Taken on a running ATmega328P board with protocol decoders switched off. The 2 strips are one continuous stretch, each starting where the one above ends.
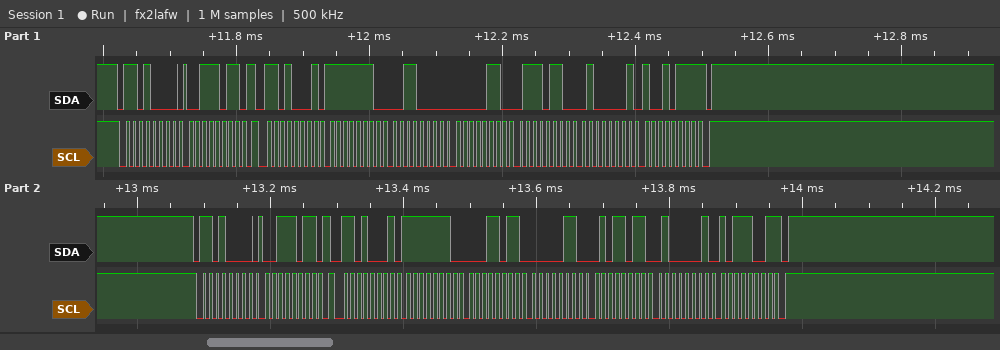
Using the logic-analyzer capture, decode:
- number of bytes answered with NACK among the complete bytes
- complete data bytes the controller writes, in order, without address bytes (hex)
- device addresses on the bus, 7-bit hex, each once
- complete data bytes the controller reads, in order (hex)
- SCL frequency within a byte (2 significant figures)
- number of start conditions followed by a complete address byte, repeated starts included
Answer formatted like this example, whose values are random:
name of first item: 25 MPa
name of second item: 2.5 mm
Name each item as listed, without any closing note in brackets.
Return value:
number of bytes answered with NACK among the complete bytes: 2
complete data bytes the controller writes, in order, without address bytes: 3B 3B
device addresses on the bus, 7-bit hex, each once: 0x68
complete data bytes the controller reads, in order: FE 30 06 76 41 97 FE 1B 06 5B 41 B9
SCL frequency within a byte: 100 kHz
number of start conditions followed by a complete address byte, repeated starts included: 4
